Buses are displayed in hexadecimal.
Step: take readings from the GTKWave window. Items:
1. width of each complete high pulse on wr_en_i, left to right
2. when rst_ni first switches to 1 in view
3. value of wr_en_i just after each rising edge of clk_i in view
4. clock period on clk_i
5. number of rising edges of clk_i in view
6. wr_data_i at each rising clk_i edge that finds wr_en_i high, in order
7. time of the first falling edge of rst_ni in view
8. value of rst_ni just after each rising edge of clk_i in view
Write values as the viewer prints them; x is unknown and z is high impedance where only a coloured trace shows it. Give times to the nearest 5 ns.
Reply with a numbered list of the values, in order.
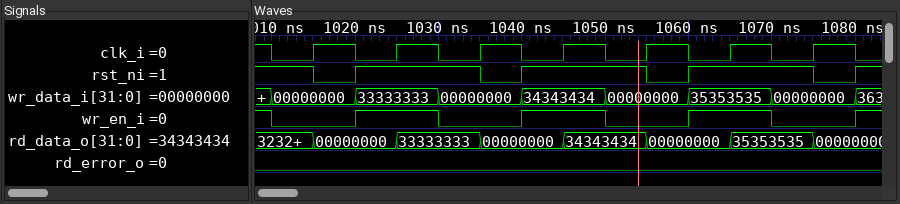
1. 10 ns, 10 ns, 10 ns
2. 1020 ns
3. 0 1 0 1 0 1 0
4. 10 ns
5. 7
6. 33333333, 34343434, 35353535
7. 1015 ns
8. 0 1 0 1 0 1 0
